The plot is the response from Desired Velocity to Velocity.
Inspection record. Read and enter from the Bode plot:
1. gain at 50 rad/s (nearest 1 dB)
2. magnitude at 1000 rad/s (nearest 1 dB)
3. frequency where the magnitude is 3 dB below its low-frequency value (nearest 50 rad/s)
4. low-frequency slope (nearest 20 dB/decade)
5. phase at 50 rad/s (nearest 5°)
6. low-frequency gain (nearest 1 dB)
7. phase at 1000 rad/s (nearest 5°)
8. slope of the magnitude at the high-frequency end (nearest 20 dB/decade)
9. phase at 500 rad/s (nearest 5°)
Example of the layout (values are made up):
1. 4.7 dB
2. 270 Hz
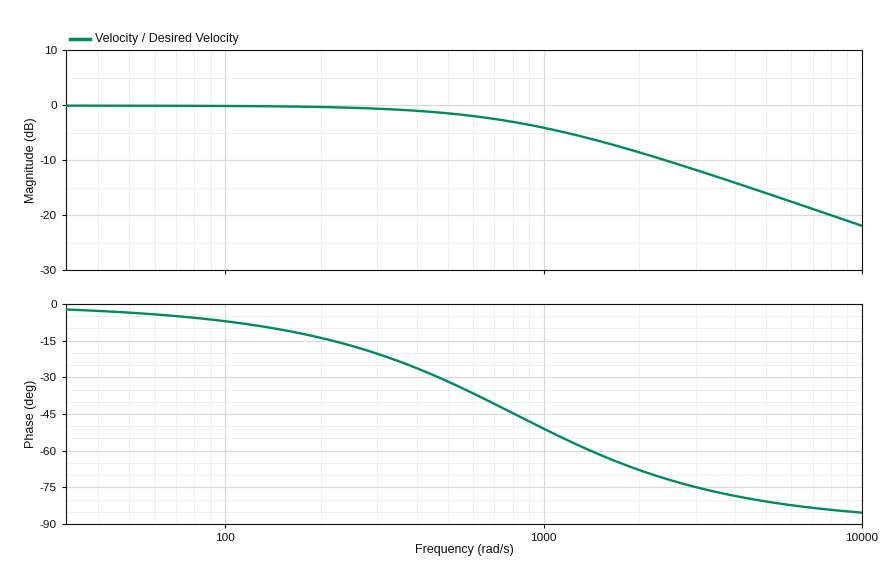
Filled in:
1. 0 dB
2. -4 dB
3. 800 rad/s
4. 0 dB/decade
5. -5°
6. 0 dB
7. -50°
8. -20 dB/decade
9. -30°
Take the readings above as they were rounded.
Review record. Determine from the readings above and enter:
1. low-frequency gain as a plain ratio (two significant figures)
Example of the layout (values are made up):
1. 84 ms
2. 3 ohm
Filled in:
1. 1.0
